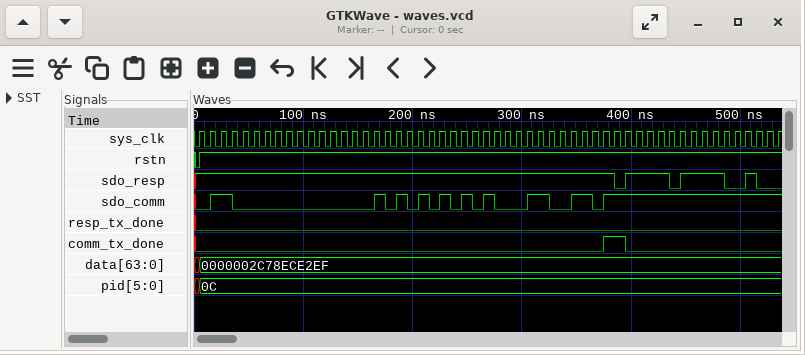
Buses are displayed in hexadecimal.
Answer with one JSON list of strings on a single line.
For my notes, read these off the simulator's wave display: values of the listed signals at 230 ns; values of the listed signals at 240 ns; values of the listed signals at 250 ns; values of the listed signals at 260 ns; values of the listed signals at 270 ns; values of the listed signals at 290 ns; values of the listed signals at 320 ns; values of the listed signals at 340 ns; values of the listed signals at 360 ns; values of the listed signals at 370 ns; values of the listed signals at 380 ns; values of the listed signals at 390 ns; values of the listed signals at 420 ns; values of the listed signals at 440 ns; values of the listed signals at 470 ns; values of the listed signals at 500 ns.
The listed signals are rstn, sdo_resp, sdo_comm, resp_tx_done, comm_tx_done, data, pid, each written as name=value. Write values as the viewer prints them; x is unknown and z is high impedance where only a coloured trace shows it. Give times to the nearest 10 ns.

["rstn=1, sdo_resp=1, sdo_comm=1, resp_tx_done=0, comm_tx_done=0, data=0000002C78ECE2EF, pid=0C", "rstn=1, sdo_resp=1, sdo_comm=0, resp_tx_done=0, comm_tx_done=0, data=0000002C78ECE2EF, pid=0C", "rstn=1, sdo_resp=1, sdo_comm=1, resp_tx_done=0, comm_tx_done=0, data=0000002C78ECE2EF, pid=0C", "rstn=1, sdo_resp=1, sdo_comm=0, resp_tx_done=0, comm_tx_done=0, data=0000002C78ECE2EF, pid=0C", "rstn=1, sdo_resp=1, sdo_comm=1, resp_tx_done=0, comm_tx_done=0, data=0000002C78ECE2EF, pid=0C", "rstn=1, sdo_resp=1, sdo_comm=0, resp_tx_done=0, comm_tx_done=0, data=0000002C78ECE2EF, pid=0C", "rstn=1, sdo_resp=1, sdo_comm=1, resp_tx_done=0, comm_tx_done=0, data=0000002C78ECE2EF, pid=0C", "rstn=1, sdo_resp=1, sdo_comm=0, resp_tx_done=0, comm_tx_done=0, data=0000002C78ECE2EF, pid=0C", "rstn=1, sdo_resp=1, sdo_comm=1, resp_tx_done=0, comm_tx_done=0, data=0000002C78ECE2EF, pid=0C", "rstn=1, sdo_resp=1, sdo_comm=0, resp_tx_done=0, comm_tx_done=0, data=0000002C78ECE2EF, pid=0C", "rstn=1, sdo_resp=1, sdo_comm=1, resp_tx_done=0, comm_tx_done=1, data=0000002C78ECE2EF, pid=0C", "rstn=1, sdo_resp=0, sdo_comm=1, resp_tx_done=0, comm_tx_done=1, data=0000002C78ECE2EF, pid=0C", "rstn=1, sdo_resp=1, sdo_comm=1, resp_tx_done=0, comm_tx_done=0, data=0000002C78ECE2EF, pid=0C", "rstn=1, sdo_resp=0, sdo_comm=1, resp_tx_done=0, comm_tx_done=0, data=0000002C78ECE2EF, pid=0C", "rstn=1, sdo_resp=1, sdo_comm=1, resp_tx_done=0, comm_tx_done=0, data=0000002C78ECE2EF, pid=0C", "rstn=1, sdo_resp=0, sdo_comm=1, resp_tx_done=0, comm_tx_done=0, data=0000002C78ECE2EF, pid=0C"]
